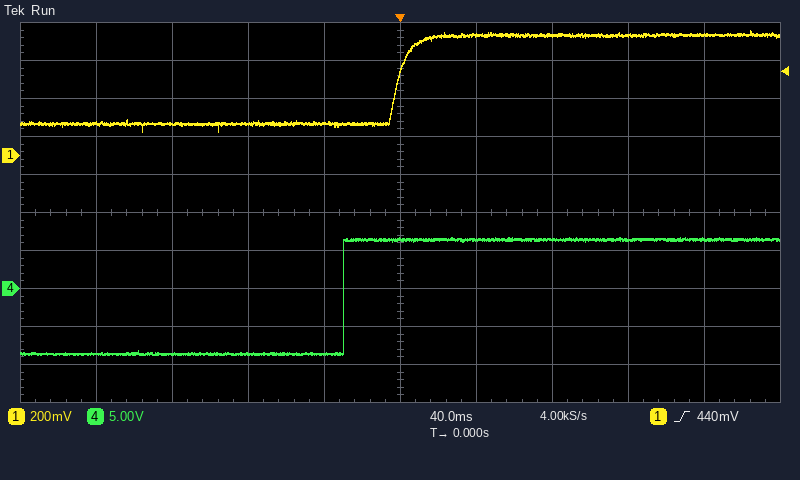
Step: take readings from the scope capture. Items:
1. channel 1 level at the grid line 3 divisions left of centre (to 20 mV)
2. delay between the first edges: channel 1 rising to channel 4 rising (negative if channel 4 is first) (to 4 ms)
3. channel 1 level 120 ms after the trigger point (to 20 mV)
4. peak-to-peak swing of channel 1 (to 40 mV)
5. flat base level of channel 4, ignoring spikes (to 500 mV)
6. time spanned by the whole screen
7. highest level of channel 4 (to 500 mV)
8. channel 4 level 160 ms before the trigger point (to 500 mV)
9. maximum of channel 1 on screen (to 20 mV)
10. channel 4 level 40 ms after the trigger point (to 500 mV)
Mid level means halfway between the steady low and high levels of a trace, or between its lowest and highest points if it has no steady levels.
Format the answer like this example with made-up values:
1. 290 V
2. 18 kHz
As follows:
1. 160 mV
2. -28 ms
3. 640 mV
4. 520 mV
5. -8.5 V
6. 400 ms
7. 6.5 V
8. -8.5 V
9. 660 mV
10. 6.5 V
